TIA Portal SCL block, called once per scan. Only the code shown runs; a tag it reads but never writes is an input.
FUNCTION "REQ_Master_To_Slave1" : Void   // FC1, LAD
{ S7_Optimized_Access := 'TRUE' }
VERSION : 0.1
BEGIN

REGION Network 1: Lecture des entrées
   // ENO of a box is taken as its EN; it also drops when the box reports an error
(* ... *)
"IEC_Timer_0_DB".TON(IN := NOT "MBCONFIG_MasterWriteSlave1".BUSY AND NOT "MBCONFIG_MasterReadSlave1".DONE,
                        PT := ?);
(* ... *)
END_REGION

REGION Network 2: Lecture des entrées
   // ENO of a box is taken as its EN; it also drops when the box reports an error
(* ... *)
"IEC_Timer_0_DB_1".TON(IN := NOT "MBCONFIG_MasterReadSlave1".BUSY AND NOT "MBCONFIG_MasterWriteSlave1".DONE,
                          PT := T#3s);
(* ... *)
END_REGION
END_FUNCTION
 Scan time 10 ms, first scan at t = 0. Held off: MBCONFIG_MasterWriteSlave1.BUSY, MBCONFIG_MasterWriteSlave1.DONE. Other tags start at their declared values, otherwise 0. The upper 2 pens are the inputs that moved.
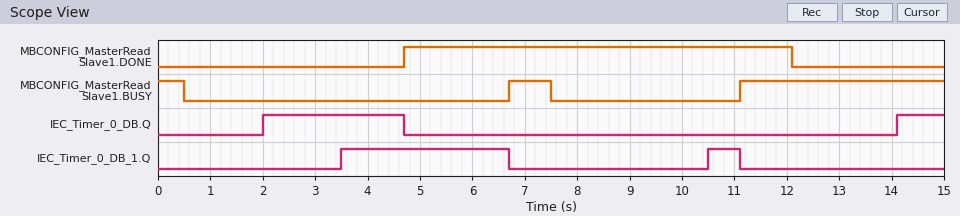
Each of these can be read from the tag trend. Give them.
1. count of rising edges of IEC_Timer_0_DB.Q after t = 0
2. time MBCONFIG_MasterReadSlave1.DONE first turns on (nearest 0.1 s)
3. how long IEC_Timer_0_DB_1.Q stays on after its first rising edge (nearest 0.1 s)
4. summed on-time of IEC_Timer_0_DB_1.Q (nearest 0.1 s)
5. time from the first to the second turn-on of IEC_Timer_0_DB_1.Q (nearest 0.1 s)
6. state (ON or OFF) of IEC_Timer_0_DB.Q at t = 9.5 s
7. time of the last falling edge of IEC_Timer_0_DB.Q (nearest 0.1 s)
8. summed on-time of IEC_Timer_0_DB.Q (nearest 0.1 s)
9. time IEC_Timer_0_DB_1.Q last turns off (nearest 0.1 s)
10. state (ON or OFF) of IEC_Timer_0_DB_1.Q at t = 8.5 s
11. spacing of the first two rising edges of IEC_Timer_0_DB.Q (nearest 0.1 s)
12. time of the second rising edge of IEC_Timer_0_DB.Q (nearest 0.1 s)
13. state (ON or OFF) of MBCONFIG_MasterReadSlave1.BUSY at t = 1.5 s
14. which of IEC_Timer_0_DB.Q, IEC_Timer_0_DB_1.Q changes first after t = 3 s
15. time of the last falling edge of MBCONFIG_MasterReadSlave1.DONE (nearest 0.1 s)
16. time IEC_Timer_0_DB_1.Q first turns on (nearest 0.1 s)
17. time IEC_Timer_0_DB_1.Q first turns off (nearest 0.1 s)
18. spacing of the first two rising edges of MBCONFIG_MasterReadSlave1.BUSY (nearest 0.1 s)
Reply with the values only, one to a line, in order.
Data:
2
4.7 s
3.2 s
3.8 s
7.0 s
OFF
4.7 s
3.6 s
11.1 s
OFF
12.1 s
14.1 s
OFF
IEC_Timer_0_DB_1.Q
12.1 s
3.5 s
6.7 s
4.4 s
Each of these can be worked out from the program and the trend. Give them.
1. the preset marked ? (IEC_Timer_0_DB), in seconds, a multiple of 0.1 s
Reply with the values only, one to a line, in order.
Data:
2.0 s
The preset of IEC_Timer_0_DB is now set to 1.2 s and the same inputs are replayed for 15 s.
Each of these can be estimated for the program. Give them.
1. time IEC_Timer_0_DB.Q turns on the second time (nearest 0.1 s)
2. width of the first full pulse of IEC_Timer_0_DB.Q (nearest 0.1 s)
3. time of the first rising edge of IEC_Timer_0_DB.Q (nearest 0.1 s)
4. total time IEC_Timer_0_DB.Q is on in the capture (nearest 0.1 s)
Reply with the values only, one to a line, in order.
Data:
13.3 s
3.5 s
1.2 s
5.2 s
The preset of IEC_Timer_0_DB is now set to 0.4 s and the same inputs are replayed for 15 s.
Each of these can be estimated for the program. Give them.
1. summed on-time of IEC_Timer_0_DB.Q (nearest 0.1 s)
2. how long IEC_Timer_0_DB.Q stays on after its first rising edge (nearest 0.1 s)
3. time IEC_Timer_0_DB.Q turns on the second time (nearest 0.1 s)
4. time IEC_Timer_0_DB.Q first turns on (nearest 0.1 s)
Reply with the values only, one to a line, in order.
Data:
6.8 s
4.3 s
12.5 s
0.4 s
